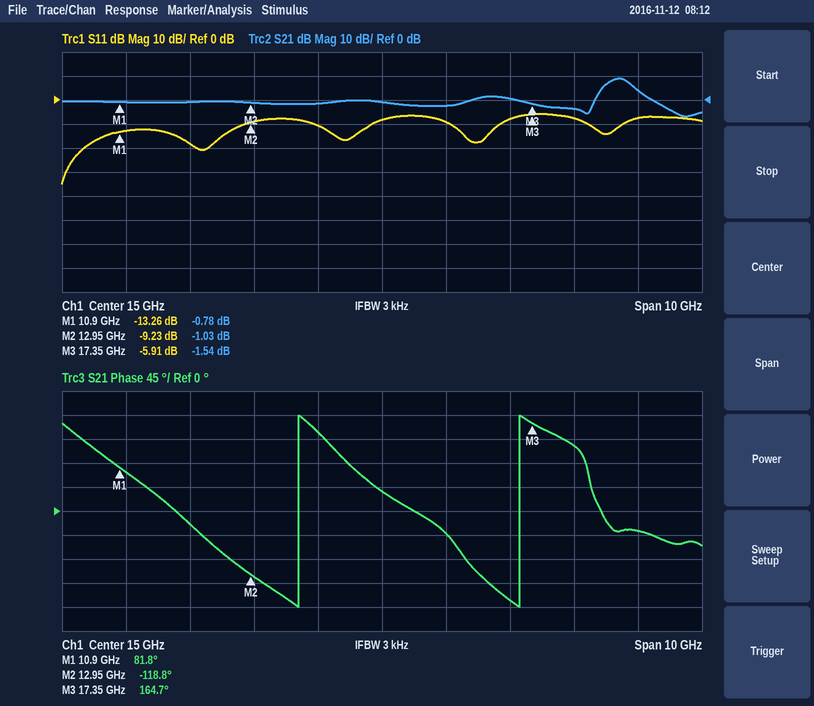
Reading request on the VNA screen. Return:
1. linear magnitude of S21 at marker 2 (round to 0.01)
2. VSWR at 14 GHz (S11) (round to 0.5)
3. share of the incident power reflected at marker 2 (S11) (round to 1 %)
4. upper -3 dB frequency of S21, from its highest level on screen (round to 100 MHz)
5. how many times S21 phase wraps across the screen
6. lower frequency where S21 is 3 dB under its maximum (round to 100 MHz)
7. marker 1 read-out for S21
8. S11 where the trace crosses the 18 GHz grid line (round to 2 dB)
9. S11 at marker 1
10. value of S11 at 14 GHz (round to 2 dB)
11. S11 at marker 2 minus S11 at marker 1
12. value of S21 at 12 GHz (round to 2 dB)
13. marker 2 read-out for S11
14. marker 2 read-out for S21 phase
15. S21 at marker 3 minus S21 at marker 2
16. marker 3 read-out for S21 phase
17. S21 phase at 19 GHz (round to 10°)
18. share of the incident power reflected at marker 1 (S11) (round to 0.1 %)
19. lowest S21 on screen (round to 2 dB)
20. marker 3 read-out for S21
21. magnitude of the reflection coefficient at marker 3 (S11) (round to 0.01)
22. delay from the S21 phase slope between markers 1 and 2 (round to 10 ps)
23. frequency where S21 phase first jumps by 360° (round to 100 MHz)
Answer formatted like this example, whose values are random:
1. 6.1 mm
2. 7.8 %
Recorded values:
1. 0.89
2. 2.0
3. 12 %
4. 18.9 GHz
5. 2
6. 18.5 GHz
7. -0.78 dB
8. -8 dB
9. -13.26 dB
10. -10 dB
11. 4.03 dB
12. 0 dB
13. -9.23 dB
14. -118.8°
15. -0.51 dB
16. 164.7°
17. -40°
18. 4.7 %
19. -6 dB
20. -1.54 dB
21. 0.51
22. 270 ps
23. 13.7 GHz
